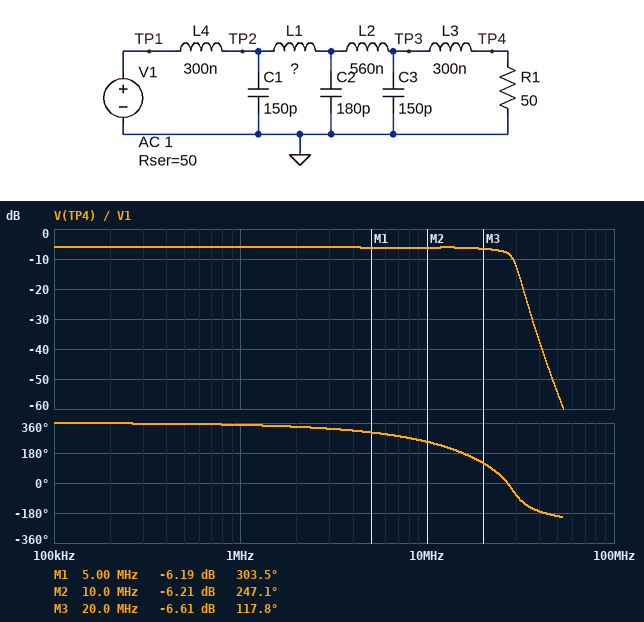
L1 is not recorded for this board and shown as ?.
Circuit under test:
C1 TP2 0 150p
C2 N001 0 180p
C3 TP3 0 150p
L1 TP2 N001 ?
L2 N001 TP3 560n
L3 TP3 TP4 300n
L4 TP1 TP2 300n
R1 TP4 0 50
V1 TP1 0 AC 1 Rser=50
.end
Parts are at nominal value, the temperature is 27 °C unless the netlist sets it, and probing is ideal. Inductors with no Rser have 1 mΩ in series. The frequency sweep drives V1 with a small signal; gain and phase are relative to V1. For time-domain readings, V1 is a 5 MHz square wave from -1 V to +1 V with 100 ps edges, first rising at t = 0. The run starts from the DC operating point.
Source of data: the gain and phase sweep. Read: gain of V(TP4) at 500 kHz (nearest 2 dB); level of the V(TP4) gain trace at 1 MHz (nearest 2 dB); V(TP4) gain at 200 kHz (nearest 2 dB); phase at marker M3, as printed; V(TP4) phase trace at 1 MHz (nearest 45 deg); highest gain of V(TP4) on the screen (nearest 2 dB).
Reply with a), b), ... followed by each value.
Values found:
a) -6 dB
b) -6 dB
c) -6 dB
d) 117.8 deg
e) 360 deg
f) -6 dB
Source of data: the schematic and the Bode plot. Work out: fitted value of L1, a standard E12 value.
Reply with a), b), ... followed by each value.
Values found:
a) 820 nH
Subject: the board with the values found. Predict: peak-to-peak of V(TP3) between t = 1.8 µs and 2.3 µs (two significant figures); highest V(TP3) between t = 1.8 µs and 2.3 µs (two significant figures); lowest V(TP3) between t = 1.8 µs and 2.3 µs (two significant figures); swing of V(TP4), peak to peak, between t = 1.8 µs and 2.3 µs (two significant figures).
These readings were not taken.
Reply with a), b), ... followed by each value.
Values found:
a) 1.5 V
b) 740 mV
c) -740 mV
d) 1.3 V
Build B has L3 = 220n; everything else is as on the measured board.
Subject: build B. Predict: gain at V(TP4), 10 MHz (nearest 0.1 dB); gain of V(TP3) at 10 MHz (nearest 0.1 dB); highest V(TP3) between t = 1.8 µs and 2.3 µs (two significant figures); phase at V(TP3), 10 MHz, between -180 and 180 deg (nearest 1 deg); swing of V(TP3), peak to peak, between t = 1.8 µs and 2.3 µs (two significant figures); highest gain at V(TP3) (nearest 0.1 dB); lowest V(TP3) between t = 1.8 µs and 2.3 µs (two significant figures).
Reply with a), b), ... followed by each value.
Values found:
a) -6.3 dB
b) -6.0 dB
c) 700 mV
d) -95 deg
e) 1.4 V
f) -5.1 dB
g) -700 mV
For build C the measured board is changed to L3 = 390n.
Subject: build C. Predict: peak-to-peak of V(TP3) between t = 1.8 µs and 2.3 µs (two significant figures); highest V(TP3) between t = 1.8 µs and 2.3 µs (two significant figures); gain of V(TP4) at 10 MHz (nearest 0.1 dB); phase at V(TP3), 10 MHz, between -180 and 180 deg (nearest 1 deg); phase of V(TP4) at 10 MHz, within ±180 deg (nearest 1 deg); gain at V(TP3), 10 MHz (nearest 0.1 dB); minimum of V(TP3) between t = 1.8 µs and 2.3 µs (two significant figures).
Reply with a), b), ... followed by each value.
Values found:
a) 1.6 V
b) 780 mV
c) -6.1 dB
d) -90 deg
e) -116 deg
f) -5.2 dB
g) -780 mV
